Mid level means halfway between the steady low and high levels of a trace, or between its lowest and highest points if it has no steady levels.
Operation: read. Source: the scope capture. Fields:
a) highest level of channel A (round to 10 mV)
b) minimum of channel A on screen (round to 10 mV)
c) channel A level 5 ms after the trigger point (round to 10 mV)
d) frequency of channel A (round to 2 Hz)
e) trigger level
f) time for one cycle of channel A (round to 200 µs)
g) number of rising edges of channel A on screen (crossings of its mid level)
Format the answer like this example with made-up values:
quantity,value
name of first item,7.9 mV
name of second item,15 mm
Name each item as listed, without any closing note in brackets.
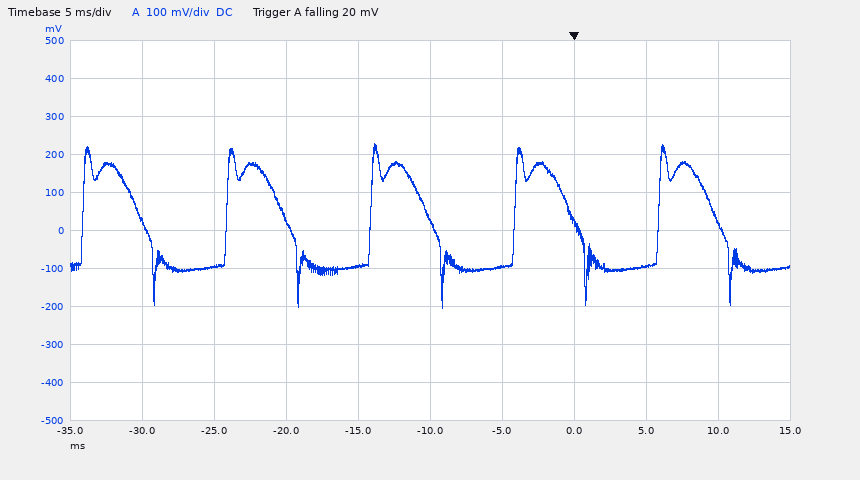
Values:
quantity,value
highest level of channel A,230 mV
minimum of channel A on screen,-210 mV
channel A level 5 ms after the trigger point,-90 mV
frequency of channel A,100 Hz
trigger level,20 mV
time for one cycle of channel A,10.0 ms
number of rising edges of channel A on screen,5
